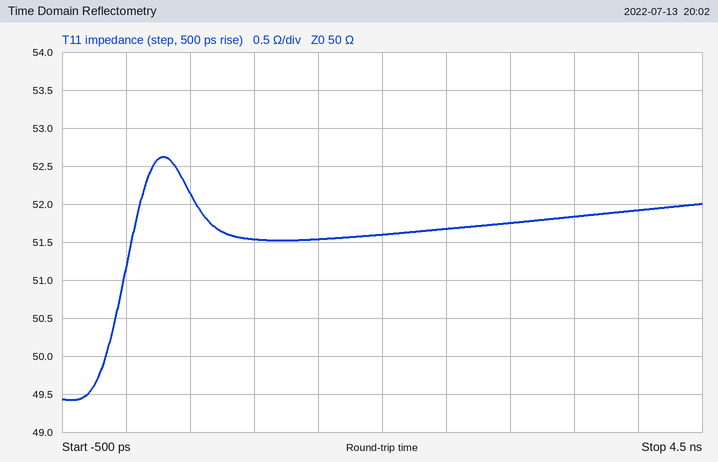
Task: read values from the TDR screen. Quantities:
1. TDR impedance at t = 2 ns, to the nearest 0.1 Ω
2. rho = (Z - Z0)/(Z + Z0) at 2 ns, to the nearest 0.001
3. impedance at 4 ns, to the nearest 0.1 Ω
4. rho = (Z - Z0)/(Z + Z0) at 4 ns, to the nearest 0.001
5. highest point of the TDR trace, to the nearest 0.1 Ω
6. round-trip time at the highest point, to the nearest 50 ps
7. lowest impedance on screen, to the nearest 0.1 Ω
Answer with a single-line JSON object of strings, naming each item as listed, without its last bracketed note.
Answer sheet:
{"TDR impedance at t = 2 ns, to the nearest 0.1 Ω": "51.6 Ω", "rho = (Z - Z0)/(Z + Z0) at 2 ns, to the nearest 0.001": "+0.016", "impedance at 4 ns, to the nearest 0.1 Ω": "51.9 Ω", "rho = (Z - Z0)/(Z + Z0) at 4 ns, to the nearest 0.001": "+0.019", "highest point of the TDR trace, to the nearest 0.1 Ω": "52.6 Ω", "round-trip time at the highest point, to the nearest 50 ps": "300 ps", "lowest impedance on screen, to the nearest 0.1 Ω": "49.4 Ω"}
